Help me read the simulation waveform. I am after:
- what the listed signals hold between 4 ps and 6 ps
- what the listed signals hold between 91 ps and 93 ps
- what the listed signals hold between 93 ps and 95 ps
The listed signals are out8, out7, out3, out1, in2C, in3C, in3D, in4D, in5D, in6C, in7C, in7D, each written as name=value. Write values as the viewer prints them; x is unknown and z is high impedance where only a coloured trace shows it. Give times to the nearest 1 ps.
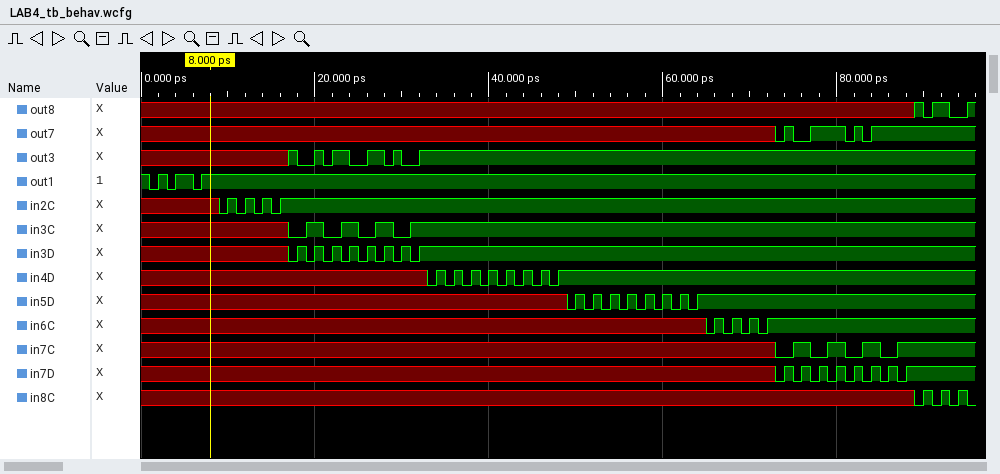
out8=x, out7=x, out3=x, out1=1, in2C=x, in3C=x, in3D=x, in4D=x, in5D=x, in6C=x, in7C=x, in7D=x
out8=1, out7=1, out3=1, out1=1, in2C=1, in3C=1, in3D=1, in4D=1, in5D=1, in6C=1, in7C=1, in7D=1
out8=0, out7=1, out3=1, out1=1, in2C=1, in3C=1, in3D=1, in4D=1, in5D=1, in6C=1, in7C=1, in7D=1
